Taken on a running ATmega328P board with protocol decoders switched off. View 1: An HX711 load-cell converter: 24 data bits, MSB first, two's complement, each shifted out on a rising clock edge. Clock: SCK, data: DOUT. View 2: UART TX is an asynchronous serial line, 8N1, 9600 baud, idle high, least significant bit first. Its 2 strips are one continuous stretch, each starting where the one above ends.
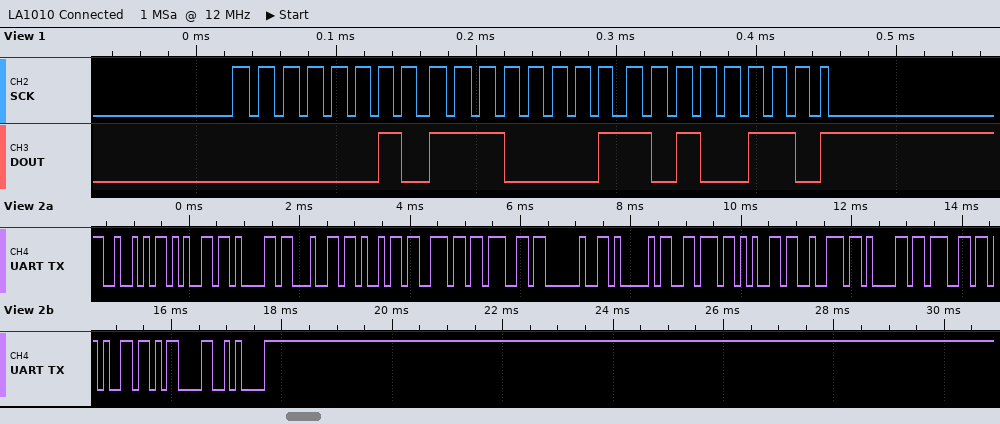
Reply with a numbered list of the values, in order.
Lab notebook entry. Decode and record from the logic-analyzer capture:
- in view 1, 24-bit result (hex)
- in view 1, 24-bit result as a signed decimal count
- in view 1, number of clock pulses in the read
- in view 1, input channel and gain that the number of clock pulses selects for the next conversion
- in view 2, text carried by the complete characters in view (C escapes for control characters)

1. 0x02E1A6
2. 188838
3. 25
4. channel A, gain 128
5. "Reading Average\r\n"
